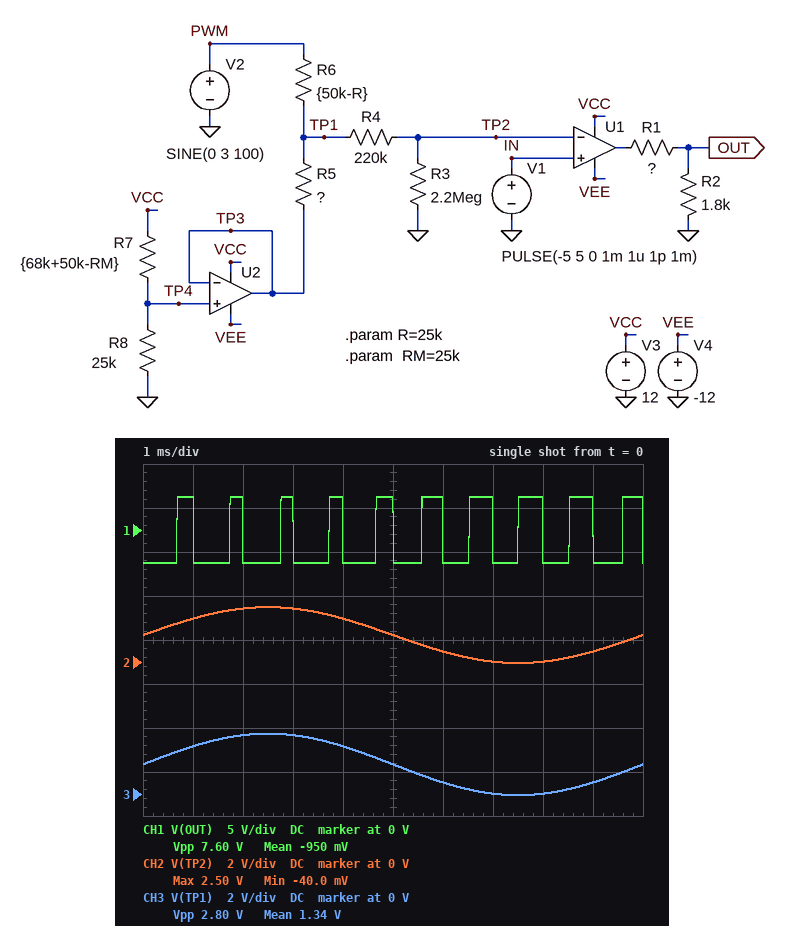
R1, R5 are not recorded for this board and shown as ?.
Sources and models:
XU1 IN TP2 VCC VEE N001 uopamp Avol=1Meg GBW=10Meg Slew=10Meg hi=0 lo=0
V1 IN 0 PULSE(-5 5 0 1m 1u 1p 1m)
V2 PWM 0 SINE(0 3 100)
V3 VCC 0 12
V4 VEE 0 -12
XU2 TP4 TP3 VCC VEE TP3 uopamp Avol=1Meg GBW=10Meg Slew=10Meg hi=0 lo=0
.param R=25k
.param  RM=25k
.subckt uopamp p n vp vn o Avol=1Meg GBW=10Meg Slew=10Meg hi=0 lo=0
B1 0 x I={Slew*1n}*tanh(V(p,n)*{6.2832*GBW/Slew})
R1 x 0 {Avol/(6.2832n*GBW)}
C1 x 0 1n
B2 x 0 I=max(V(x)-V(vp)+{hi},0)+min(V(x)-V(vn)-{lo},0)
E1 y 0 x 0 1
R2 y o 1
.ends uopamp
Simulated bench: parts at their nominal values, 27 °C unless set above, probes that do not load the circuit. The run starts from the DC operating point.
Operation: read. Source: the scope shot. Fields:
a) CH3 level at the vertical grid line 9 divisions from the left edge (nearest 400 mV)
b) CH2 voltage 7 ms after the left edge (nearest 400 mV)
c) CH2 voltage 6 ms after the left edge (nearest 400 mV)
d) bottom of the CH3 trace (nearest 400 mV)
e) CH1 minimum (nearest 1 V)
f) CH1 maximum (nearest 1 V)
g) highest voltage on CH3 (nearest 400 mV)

400 mV
0 V
400 mV
0 V
-4 V
4 V
2.8 V
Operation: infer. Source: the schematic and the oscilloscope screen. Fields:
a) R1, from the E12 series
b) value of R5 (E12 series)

3.9 kΩ
22 kΩ
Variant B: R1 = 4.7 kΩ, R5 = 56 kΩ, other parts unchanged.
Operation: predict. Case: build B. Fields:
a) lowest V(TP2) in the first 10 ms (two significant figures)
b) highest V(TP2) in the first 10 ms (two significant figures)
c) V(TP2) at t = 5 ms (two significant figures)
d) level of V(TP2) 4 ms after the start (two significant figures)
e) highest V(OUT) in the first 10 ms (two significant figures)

-1.2 V
2.6 V
710 mV
1.8 V
3.3 V
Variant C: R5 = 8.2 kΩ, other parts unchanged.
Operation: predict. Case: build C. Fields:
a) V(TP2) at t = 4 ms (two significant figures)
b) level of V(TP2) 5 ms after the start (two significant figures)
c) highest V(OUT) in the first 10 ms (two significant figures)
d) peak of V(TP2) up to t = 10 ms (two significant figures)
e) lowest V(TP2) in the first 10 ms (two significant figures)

2.1 V
1.7 V
3.8 V
2.4 V
1.1 V
